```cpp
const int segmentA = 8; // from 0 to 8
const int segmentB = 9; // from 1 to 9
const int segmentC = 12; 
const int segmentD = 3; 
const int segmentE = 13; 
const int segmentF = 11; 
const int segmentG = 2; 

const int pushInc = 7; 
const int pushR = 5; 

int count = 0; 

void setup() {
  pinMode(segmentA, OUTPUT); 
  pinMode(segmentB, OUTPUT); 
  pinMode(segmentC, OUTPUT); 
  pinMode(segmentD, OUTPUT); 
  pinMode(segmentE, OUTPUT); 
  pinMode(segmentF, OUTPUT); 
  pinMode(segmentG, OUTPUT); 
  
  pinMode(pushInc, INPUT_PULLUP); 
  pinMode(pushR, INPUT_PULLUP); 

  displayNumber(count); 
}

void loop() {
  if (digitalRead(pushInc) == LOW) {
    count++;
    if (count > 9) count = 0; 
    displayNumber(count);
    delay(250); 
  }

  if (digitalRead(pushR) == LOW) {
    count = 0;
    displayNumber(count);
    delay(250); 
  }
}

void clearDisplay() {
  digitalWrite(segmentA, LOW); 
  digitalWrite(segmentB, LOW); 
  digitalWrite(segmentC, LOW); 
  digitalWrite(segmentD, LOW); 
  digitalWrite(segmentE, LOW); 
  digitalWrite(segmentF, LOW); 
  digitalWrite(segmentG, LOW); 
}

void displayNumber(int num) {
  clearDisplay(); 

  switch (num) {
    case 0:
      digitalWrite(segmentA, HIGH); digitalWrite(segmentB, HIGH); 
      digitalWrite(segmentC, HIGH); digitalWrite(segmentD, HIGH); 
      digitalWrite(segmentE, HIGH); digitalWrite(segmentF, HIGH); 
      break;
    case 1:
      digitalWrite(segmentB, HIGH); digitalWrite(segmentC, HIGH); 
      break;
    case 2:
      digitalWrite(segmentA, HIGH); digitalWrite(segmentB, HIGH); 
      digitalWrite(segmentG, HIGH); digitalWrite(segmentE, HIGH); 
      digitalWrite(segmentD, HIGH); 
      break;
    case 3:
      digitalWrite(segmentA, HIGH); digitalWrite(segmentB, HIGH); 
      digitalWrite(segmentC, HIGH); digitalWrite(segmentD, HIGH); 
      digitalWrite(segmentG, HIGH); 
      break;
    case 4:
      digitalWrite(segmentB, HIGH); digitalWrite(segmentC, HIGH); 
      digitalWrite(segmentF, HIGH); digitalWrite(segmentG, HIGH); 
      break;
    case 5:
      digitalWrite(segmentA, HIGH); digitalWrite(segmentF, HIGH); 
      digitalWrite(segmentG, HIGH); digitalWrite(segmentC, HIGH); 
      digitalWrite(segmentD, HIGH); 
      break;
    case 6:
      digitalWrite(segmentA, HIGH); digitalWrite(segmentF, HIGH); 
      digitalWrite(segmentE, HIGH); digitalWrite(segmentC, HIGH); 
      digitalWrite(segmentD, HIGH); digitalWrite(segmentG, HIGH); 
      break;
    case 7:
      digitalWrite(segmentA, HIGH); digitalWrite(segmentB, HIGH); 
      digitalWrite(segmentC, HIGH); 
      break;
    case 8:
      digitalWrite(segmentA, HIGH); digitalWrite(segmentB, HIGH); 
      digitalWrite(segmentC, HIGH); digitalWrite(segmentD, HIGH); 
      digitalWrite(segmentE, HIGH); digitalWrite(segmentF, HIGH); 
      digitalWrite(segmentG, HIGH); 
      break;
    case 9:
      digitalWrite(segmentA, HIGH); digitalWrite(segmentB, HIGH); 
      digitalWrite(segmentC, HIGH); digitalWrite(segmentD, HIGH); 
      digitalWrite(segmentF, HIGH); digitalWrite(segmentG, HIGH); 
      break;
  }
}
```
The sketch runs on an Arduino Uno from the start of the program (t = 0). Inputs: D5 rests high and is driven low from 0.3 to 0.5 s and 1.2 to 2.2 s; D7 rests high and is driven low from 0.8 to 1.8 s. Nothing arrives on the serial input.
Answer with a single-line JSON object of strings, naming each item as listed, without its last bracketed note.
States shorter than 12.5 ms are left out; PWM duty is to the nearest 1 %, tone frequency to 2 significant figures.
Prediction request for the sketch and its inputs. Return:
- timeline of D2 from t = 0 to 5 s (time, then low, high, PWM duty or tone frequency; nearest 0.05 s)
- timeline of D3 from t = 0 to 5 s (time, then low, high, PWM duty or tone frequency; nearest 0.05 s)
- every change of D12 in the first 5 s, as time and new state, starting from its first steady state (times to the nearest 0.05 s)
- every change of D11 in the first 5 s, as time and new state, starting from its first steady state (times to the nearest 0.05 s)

{"timeline of D2 from t = 0 to 5 s": "0 s low; 1.05 s high; 1.3 s low", "timeline of D3 from t = 0 to 5 s": "0 s high; 0.8 s low; 1.05 s high; 1.55 s low; 1.8 s high", "every change of D12 in the first 5 s, as time and new state, starting from its first steady state": "0 s high; 1.05 s low; 1.3 s high", "every change of D11 in the first 5 s, as time and new state, starting from its first steady state": "0 s high; 0.8 s low; 1.3 s high; 1.55 s low; 1.8 s high"}
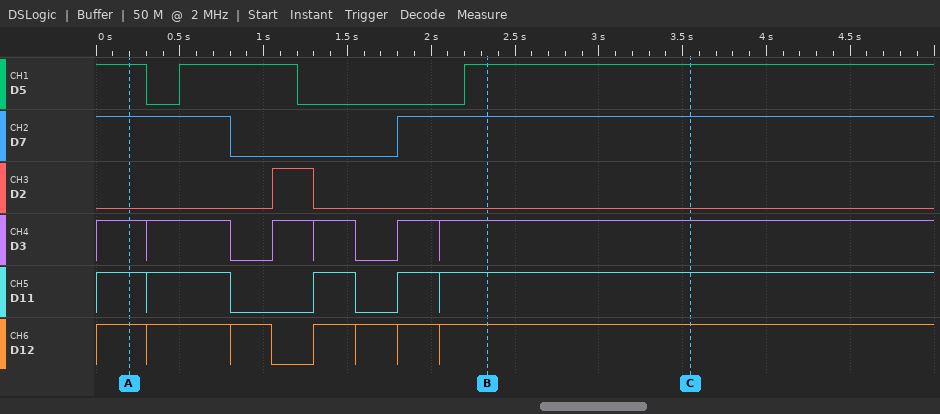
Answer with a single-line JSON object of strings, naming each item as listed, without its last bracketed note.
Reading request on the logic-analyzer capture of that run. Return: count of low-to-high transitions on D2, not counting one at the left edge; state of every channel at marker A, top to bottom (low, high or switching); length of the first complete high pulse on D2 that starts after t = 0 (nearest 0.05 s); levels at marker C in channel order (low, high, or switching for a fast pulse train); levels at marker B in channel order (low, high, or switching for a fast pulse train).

{"count of low-to-high transitions on D2, not counting one at the left edge": "1", "state of every channel at marker A, top to bottom": "D5 high, D7 high, D2 low, D3 high, D11 high, D12 high", "length of the first complete high pulse on D2 that starts after t = 0": "0.25 s", "levels at marker C in channel order": "D5 high, D7 high, D2 low, D3 high, D11 high, D12 high", "levels at marker B in channel order": "D5 high, D7 high, D2 low, D3 high, D11 high, D12 high"}
